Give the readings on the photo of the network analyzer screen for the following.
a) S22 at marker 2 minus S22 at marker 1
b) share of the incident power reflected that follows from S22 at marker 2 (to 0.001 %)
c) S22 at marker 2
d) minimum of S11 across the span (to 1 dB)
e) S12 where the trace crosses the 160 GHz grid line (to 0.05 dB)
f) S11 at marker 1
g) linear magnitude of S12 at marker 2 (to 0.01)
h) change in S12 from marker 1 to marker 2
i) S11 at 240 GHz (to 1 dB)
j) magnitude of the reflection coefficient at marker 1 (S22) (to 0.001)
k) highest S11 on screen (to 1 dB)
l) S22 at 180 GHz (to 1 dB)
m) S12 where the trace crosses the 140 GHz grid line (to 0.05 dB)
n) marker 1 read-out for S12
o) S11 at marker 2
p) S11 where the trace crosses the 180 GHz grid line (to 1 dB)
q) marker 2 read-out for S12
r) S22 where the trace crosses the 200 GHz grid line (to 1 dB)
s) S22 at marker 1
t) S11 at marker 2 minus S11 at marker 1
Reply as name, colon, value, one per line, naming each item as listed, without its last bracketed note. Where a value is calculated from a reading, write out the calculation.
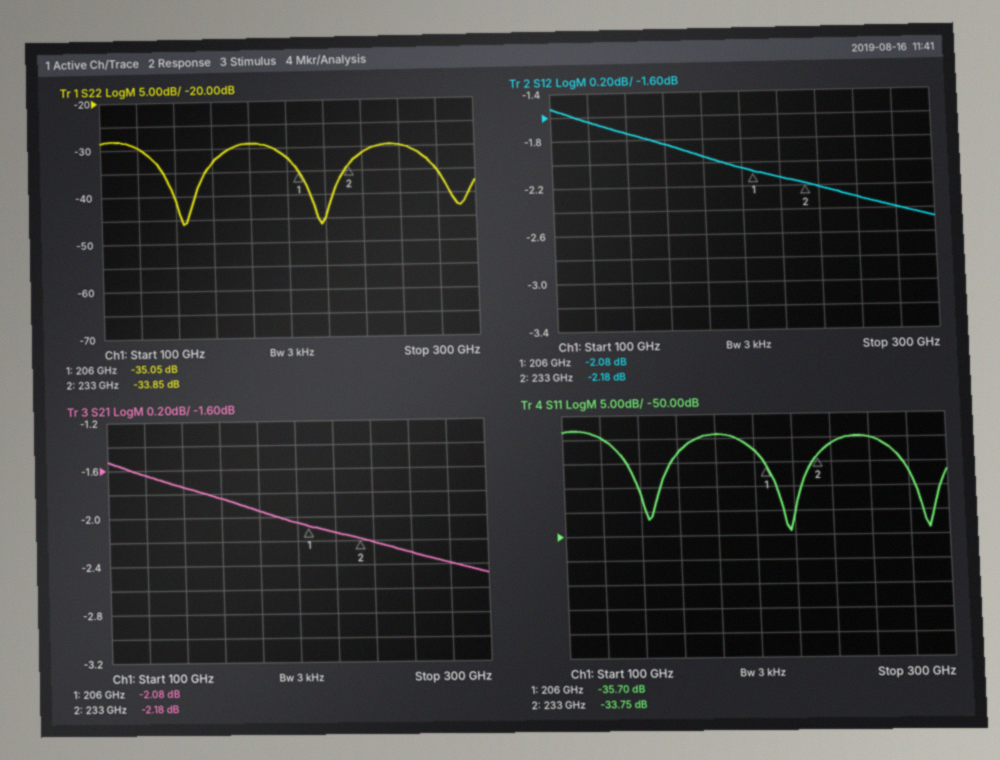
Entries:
S22 at marker 2 minus S22 at marker 1: -33.85 − (-35.05) = 1.20 dB
share of the incident power reflected that follows from S22 at marker 2: 10^(-33.85/10) ≈ 0.041 %
S22 at marker 2: -33.85 dB
minimum of S11 across the span: -49 dB
S12 where the trace crosses the 160 GHz grid line: -1.85 dB
S11 at marker 1: -35.70 dB
linear magnitude of S12 at marker 2: 10^(-2.18/20) ≈ 0.78
change in S12 from marker 1 to marker 2: -2.18 − (-2.08) = -0.10 dB
S11 at 240 GHz: -31 dB
magnitude of the reflection coefficient at marker 1 (S22): 10^(-35.05/20) ≈ 0.018
highest S11 on screen: -28 dB
S22 at 180 GHz: -29 dB
S12 where the trace crosses the 140 GHz grid line: -1.75 dB
marker 1 read-out for S12: -2.08 dB
S11 at marker 2: -33.75 dB
S11 where the trace crosses the 180 GHz grid line: -29 dB
marker 2 read-out for S12: -2.18 dB
S22 where the trace crosses the 200 GHz grid line: -32 dB
S22 at marker 1: -35.05 dB
S11 at marker 2 minus S11 at marker 1: -33.75 − (-35.7) = 1.95 dB
